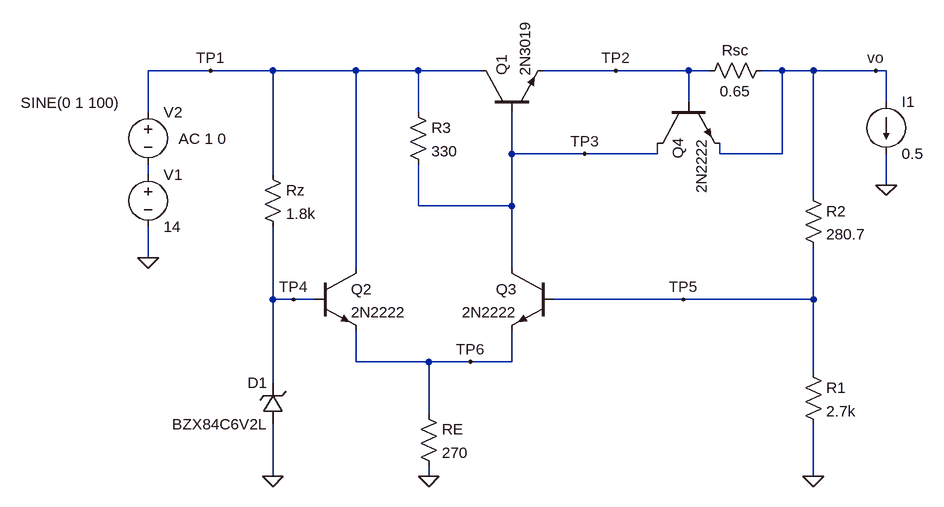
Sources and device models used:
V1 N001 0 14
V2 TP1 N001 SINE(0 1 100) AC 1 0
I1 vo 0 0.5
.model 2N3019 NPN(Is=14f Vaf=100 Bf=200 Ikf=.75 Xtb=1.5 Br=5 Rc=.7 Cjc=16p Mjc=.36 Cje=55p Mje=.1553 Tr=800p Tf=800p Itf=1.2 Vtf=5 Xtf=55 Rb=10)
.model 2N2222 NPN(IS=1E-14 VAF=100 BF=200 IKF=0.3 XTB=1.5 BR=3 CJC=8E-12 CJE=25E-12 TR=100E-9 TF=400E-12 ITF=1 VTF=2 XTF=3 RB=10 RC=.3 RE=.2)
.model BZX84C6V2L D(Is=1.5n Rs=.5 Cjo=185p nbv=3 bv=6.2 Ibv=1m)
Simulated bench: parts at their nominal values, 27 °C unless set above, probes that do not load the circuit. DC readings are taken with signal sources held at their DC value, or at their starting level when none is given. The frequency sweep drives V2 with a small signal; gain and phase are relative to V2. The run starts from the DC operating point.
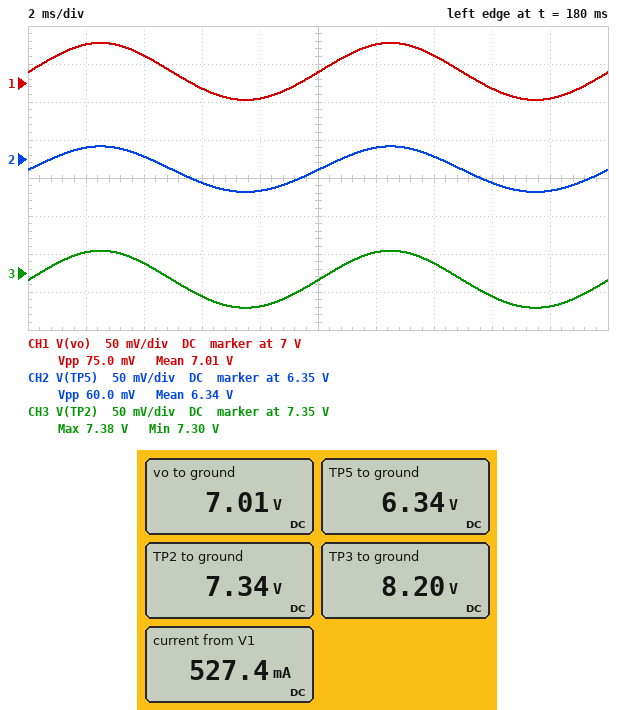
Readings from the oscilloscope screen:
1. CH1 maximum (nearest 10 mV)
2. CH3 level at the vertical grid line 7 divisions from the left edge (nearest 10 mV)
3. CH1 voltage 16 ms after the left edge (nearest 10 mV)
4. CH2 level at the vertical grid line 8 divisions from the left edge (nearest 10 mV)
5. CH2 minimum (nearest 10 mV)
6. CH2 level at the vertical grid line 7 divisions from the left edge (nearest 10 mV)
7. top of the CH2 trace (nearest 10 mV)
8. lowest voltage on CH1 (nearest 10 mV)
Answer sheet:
7.05 V
7.36 V
6.99 V
6.32 V
6.31 V
6.35 V
6.37 V
6.98 V
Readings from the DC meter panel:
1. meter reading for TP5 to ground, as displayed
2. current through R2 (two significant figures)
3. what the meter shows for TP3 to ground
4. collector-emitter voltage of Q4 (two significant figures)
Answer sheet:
6.34 V
2.4 mA
8.20 V
1.2 V
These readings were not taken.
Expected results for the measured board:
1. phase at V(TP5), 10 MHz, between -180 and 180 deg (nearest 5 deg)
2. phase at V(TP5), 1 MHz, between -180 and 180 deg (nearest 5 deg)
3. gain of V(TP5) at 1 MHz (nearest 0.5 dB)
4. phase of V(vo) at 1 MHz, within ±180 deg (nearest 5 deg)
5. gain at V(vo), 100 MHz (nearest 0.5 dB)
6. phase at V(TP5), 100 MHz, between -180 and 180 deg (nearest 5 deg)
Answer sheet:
45 deg
20 deg
-30.0 dB
25 deg
-2.5 dB
15 deg
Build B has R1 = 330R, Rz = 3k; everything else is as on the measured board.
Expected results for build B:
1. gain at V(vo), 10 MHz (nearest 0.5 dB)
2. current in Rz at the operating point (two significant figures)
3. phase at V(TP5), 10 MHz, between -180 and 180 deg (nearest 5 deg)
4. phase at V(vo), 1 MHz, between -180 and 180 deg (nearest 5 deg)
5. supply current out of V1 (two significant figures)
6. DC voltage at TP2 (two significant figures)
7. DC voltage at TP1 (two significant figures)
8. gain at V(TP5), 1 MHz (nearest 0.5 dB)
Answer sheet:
-1.0 dB
2.6 mA
-15 deg
15 deg
540 mA
12 V
14 V
-8.5 dB
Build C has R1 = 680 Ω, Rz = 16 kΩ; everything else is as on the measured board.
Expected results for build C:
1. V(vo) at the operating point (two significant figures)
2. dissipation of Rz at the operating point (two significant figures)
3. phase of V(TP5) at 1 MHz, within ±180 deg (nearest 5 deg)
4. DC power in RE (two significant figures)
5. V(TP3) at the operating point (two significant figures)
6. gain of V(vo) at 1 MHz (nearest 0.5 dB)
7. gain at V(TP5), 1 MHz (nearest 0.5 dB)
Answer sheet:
8.7 V
3.9 mW
30 deg
110 mW
9.9 V
-25.0 dB
-28.5 dB
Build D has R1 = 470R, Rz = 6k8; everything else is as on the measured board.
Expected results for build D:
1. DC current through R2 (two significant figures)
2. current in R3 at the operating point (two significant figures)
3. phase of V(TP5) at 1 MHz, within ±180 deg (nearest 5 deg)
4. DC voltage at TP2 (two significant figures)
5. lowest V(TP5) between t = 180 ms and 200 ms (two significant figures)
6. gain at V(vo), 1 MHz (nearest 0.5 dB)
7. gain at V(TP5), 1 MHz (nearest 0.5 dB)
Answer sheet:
13 mA
8.9 mA
30 deg
10 V
6.1 V
-23.0 dB
-27.5 dB
